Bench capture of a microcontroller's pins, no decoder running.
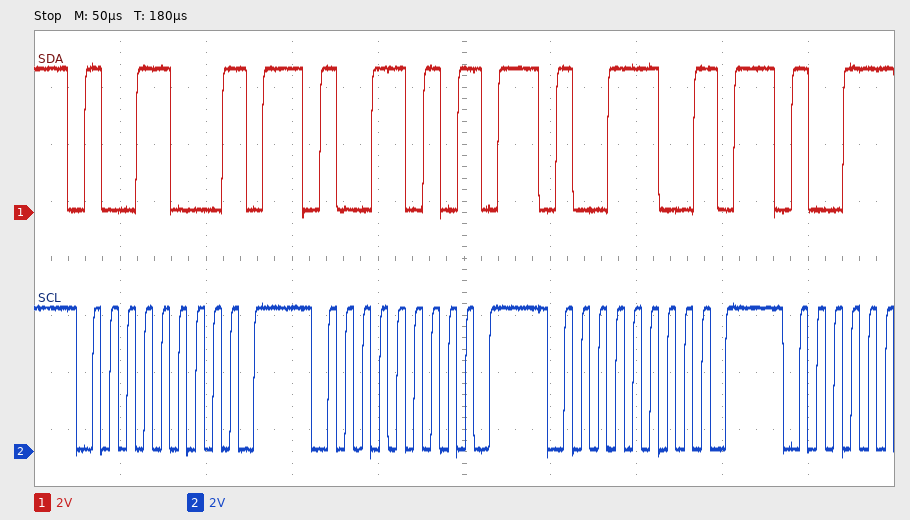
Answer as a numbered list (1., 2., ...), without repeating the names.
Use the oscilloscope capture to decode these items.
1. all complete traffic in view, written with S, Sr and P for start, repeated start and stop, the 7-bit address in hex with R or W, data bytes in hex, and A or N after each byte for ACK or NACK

1. S 4CW N P S 4DW N P S 4EW N P
